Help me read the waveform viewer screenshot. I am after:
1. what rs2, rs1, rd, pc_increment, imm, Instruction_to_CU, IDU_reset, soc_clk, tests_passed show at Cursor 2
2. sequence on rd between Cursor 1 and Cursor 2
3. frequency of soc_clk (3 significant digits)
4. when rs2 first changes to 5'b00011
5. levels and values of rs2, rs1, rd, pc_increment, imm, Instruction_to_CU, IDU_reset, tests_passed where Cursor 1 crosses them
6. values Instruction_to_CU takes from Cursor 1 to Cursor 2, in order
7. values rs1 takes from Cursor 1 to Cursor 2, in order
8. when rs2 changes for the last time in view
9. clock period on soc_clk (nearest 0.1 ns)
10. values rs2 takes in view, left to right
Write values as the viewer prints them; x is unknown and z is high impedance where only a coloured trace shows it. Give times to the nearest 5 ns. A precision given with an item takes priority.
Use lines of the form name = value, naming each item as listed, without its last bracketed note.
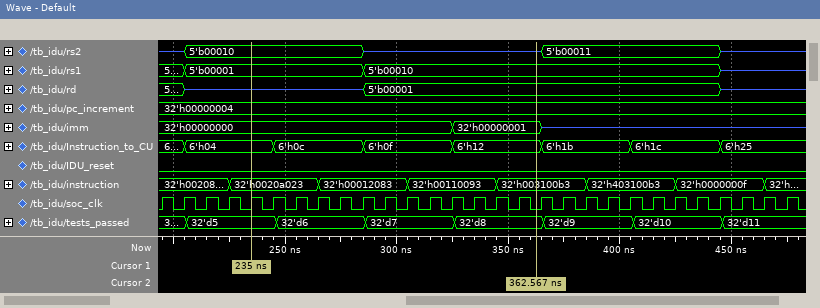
what rs2, rs1, rd, pc_increment, imm, Instruction_to_CU, IDU_reset, soc_clk, tests_passed show at Cursor 2 = rs2=z, rs1=5'b00010, rd=5'b00001, pc_increment=32'h00000004, imm=32'h00000001, Instruction_to_CU=6'h12, IDU_reset=0, soc_clk=0, tests_passed=32'd8
sequence on rd between Cursor 1 and Cursor 2 = z, 5'b00001
frequency of soc_clk = 100 MHz
when rs2 first changes to 5'b00011 = 365 ns
levels and values of rs2, rs1, rd, pc_increment, imm, Instruction_to_CU, IDU_reset, tests_passed where Cursor 1 crosses them = rs2=5'b00010, rs1=5'b00001, rd=z, pc_increment=32'h00000004, imm=32'h00000000, Instruction_to_CU=6'h04, IDU_reset=0, tests_passed=32'd5
values Instruction_to_CU takes from Cursor 1 to Cursor 2, in order = 6'h04, 6'h0c, 6'h0f, 6'h12
values rs1 takes from Cursor 1 to Cursor 2, in order = 5'b00001, 5'b00010
when rs2 changes for the last time in view = 445 ns
clock period on soc_clk = 10 ns
values rs2 takes in view, left to right = z, 5'b00010, z, 5'b00011, z
